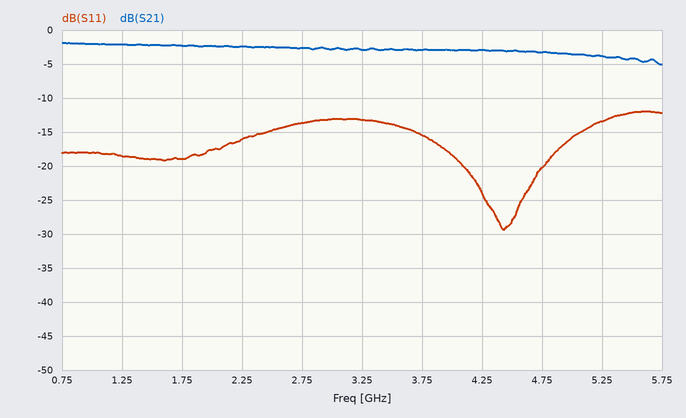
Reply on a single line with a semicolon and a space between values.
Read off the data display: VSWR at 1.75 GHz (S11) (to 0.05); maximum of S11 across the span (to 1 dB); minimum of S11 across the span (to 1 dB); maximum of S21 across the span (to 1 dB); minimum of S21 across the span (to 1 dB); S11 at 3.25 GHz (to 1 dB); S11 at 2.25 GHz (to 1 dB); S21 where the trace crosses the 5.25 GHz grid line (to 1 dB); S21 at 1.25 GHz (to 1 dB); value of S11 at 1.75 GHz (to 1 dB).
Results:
1.25; -12 dB; -29 dB; -2 dB; -5 dB; -13 dB; -16 dB; -4 dB; -2 dB; -19 dB
